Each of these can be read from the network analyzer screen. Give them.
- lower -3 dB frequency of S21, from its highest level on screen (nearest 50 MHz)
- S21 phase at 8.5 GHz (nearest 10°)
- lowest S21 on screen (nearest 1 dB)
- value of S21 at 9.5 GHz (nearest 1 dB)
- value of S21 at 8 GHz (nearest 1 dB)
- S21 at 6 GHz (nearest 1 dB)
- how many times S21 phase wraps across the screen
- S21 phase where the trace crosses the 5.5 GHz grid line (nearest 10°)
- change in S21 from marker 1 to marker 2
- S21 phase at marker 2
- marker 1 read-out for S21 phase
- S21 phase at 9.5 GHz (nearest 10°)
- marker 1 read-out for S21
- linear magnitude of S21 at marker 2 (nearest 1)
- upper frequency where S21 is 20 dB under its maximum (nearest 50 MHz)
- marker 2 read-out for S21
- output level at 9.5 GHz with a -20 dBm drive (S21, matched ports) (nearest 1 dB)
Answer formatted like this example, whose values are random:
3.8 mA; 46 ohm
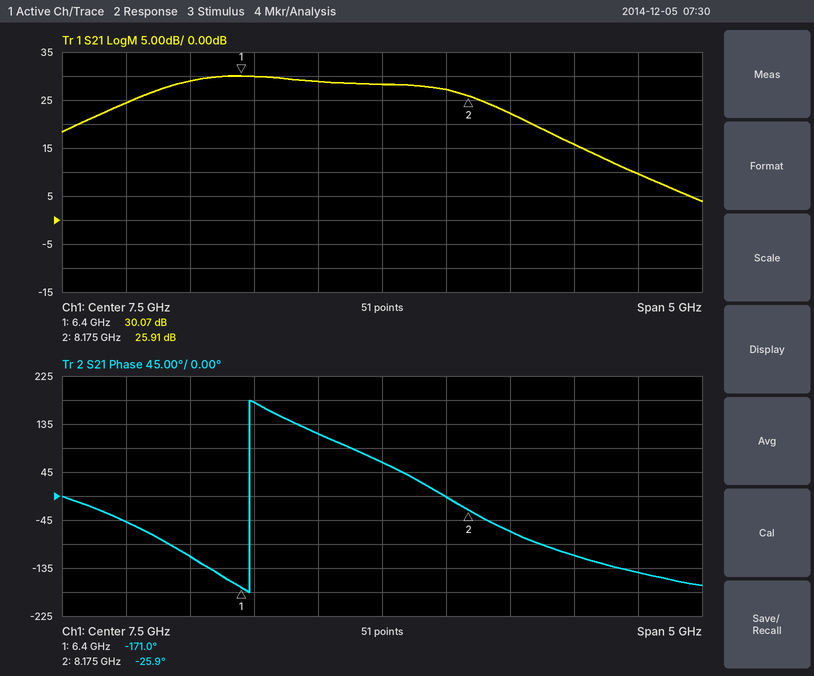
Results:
5.75 GHz; -70°; 4 dB; 10 dB; 27 dB; 29 dB; 1; -50°; -4.16 dB; -25.9°; -171.0°; -140°; 30.07 dB; 20; 9.45 GHz; 25.91 dB; -10 dBm
